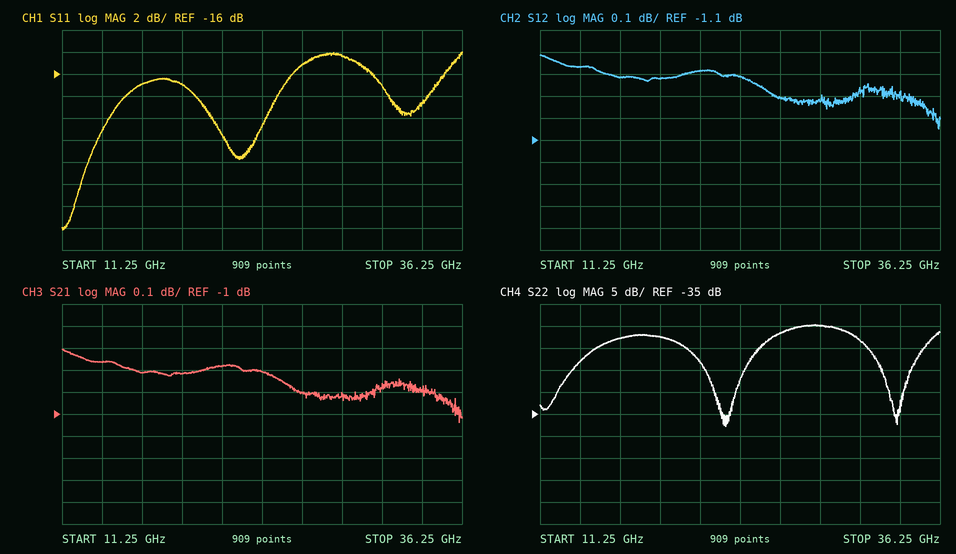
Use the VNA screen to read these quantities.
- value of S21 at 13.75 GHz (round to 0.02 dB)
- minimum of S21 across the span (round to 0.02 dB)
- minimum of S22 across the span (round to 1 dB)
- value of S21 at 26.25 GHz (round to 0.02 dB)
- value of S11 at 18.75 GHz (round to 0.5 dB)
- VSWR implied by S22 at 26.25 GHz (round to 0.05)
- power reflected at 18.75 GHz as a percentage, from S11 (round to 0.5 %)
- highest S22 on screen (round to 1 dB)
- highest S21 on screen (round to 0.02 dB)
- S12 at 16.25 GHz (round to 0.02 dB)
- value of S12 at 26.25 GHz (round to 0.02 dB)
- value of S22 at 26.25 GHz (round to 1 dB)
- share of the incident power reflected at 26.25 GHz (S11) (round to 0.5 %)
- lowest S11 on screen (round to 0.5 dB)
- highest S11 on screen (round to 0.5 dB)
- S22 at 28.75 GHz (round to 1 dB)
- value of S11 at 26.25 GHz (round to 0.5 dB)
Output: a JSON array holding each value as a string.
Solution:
["-0.76 dB", "-1.04 dB", "-38 dB", "-0.90 dB", "-17.0 dB", "1.35", "2.0 %", "-15 dB", "-0.70 dB", "-0.82 dB", "-0.90 dB", "-17 dB", "3.0 %", "-30.0 dB", "-14.0 dB", "-15 dB", "-15.0 dB"]
